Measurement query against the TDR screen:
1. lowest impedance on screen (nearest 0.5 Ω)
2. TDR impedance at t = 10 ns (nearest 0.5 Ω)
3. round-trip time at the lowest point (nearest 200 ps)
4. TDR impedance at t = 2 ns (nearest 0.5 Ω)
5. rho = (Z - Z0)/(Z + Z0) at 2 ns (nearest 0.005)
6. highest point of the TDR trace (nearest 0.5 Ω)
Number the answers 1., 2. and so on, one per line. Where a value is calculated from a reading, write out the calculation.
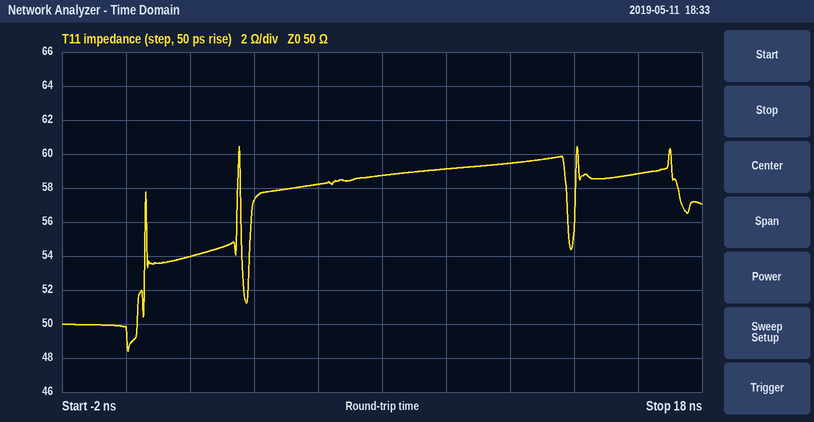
1. 48.5 Ω
2. 59.0 Ω
3. 0.0 ns
4. 54.0 Ω
5. (54 − 50)/(54 + 50) ≈ +0.0385, so +0.040 to the nearest 0.005
6. 60.5 Ω
